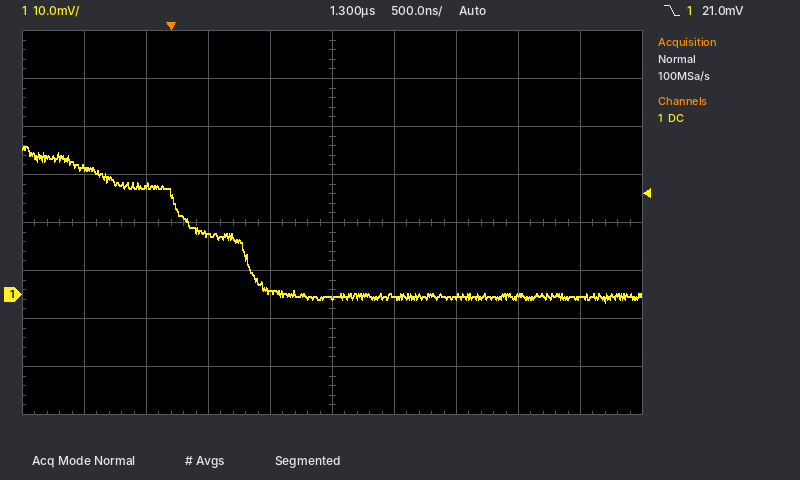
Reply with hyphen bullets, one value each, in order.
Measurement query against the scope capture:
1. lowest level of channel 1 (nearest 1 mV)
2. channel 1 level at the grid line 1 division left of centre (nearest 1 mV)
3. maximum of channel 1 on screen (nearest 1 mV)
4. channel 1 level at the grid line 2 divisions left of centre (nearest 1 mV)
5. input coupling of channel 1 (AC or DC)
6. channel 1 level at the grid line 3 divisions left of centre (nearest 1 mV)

- -2 mV
- 1 mV
- 31 mV
- 13 mV
- DC
- 23 mV
